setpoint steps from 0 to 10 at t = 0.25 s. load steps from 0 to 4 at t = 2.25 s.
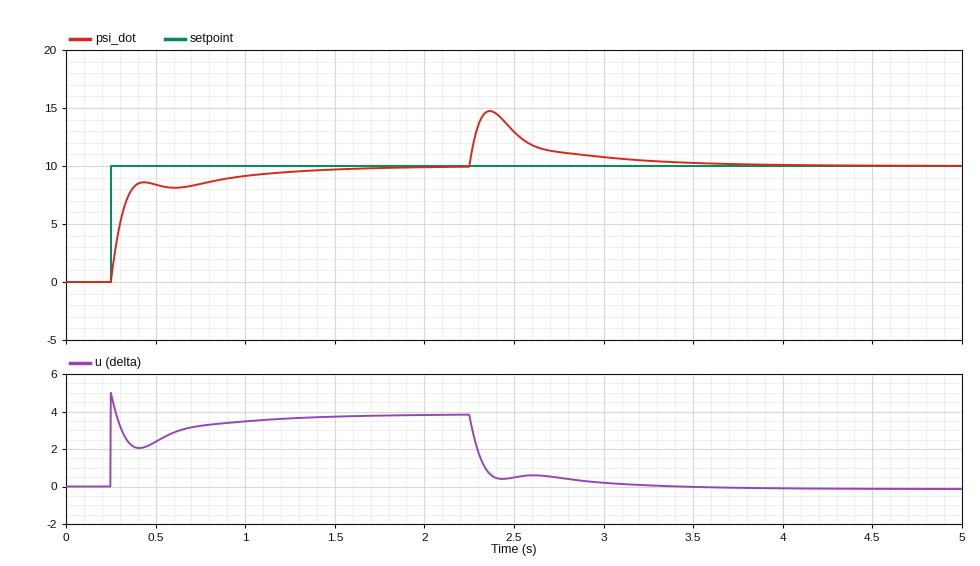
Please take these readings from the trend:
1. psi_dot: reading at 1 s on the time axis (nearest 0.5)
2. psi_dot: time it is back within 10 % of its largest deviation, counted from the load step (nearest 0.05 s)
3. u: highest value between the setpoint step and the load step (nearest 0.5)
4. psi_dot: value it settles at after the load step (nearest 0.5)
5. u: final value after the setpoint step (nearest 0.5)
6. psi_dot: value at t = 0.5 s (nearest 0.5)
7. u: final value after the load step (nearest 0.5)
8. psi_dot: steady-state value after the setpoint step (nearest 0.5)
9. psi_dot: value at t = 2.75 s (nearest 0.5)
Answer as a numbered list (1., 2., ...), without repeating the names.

1. 9.0
2. 0.95 s
3. 5.0
4. 10.0
5. 4.0
6. 8.5
7. 0.0
8. 10.0
9. 11.0
